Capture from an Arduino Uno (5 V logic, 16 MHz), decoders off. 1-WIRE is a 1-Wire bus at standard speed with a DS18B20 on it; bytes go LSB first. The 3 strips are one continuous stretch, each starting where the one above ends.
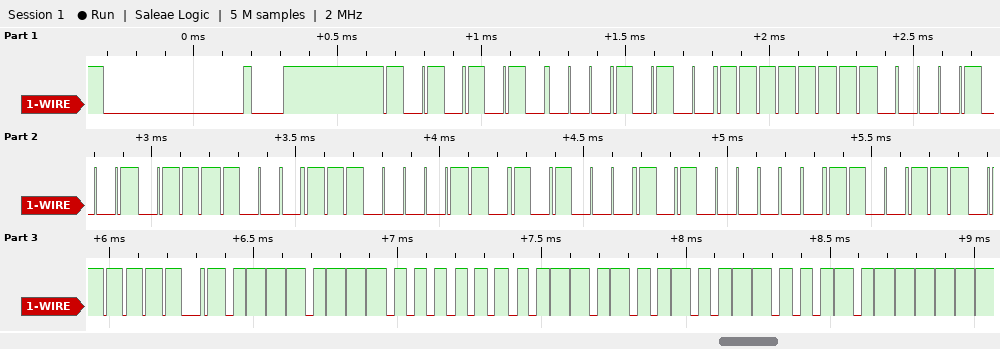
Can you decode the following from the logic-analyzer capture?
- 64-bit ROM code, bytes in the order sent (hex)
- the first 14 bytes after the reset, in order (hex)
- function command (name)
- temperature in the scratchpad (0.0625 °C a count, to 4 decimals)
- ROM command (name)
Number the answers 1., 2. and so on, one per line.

1. 28 FF 90 1E 87 15 05 E6
2. 55 28 FF 90 1E 87 15 05 E6 BE EE 00 4B 46
3. Read Scratchpad
4. 14.8750 °C
5. Match ROM
